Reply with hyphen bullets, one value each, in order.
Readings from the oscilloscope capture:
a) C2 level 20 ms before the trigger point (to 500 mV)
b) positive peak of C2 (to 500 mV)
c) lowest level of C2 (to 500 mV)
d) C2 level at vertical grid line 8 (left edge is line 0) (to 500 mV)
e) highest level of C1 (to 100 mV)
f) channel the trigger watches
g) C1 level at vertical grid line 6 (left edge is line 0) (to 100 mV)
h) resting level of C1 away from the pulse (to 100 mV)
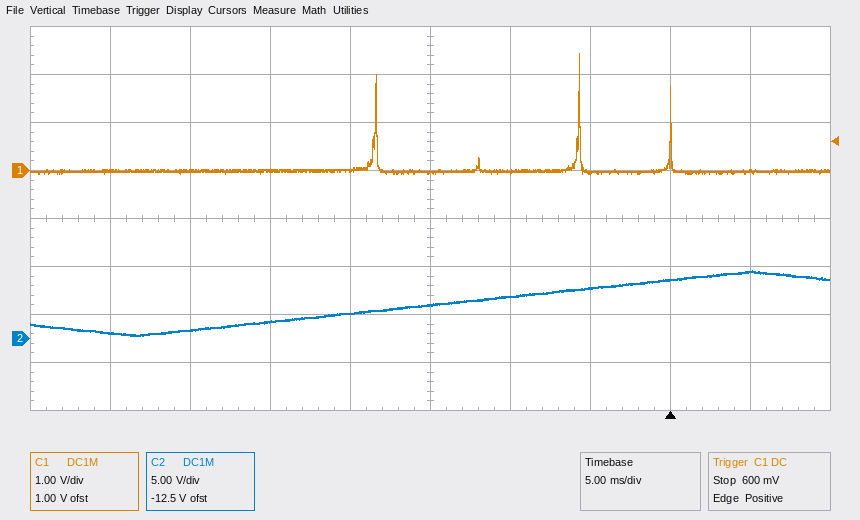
- 2.5 V
- 7.0 V
- 500 mV
- 6.0 V
- 2.4 V
- C1
- 0.0 V
- 0.0 V
